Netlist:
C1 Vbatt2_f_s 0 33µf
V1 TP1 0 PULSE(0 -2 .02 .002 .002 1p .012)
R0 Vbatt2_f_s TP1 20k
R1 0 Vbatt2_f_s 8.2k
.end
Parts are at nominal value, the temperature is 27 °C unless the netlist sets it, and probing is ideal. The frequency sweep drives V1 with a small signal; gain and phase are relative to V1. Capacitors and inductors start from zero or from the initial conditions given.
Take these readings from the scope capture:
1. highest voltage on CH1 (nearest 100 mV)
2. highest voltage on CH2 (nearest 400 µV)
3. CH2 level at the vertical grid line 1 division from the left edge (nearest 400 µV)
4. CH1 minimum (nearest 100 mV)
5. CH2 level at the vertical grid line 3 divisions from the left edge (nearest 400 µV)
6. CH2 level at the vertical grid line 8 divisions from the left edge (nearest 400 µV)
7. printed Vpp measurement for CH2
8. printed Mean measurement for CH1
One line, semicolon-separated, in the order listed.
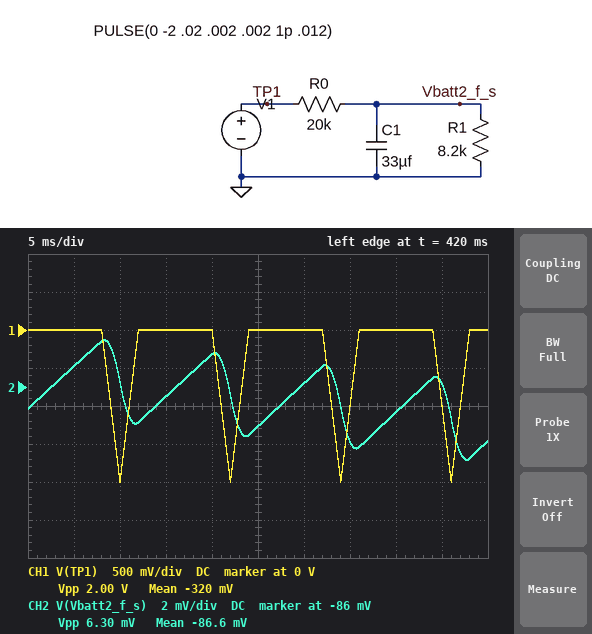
0 V; -83.6 mV; -84.8 mV; -2.0 V; -86.4 mV; -87.2 mV; 6.30 mV; -320 mV
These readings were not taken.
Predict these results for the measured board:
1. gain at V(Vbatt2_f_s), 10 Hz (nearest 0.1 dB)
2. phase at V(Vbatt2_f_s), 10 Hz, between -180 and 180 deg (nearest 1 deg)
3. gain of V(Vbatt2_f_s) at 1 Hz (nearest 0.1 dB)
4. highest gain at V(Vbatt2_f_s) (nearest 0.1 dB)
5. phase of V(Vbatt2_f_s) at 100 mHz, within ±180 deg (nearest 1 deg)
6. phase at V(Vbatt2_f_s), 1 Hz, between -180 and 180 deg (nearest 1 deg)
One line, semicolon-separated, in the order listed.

-32.4 dB; -85 deg; -14.6 dB; -10.7 dB; -7 deg; -50 deg
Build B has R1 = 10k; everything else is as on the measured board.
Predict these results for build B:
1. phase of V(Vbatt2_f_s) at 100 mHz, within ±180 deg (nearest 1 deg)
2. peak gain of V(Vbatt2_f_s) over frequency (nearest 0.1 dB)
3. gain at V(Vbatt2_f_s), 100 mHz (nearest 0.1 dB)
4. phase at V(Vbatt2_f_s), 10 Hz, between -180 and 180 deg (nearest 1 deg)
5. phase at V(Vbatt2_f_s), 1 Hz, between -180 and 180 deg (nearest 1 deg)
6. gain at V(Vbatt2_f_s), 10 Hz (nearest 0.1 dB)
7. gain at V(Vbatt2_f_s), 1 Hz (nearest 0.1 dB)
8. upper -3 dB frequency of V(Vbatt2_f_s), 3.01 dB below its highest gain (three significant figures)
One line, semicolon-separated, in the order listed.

-8 deg; -9.5 dB; -9.6 dB; -86 deg; -54 deg; -32.4 dB; -14.2 dB; 723 mHz
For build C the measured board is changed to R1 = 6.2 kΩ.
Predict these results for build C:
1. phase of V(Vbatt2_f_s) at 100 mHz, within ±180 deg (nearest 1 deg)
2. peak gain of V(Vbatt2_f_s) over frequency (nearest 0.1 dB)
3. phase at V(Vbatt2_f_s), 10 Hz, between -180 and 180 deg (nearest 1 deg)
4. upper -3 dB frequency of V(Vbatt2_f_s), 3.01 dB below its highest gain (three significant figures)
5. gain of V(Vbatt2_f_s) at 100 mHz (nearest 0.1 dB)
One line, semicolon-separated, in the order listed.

-6 deg; -12.5 dB; -84 deg; 1.02 Hz; -12.6 dB
